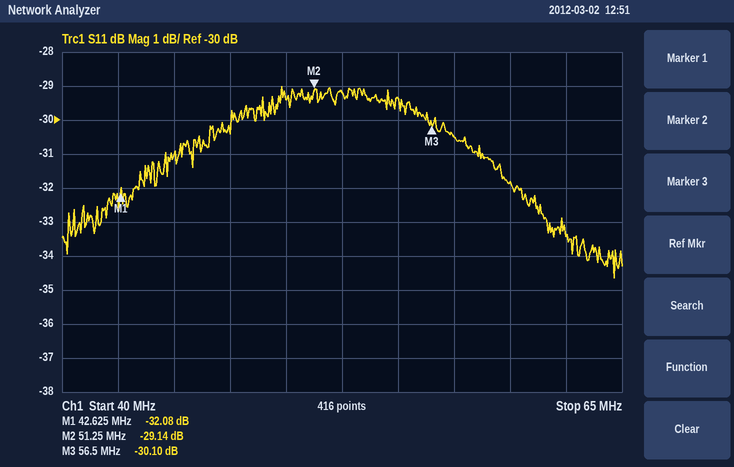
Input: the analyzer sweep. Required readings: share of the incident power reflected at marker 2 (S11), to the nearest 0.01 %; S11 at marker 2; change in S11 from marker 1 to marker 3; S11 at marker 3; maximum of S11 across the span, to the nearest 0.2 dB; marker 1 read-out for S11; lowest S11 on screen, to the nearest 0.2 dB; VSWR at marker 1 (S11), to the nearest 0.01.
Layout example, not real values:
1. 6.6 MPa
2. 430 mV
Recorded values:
1. 0.12 %
2. -29.14 dB
3. 1.98 dB
4. -30.10 dB
5. -29.0 dB
6. -32.08 dB
7. -34.6 dB
8. 1.05
